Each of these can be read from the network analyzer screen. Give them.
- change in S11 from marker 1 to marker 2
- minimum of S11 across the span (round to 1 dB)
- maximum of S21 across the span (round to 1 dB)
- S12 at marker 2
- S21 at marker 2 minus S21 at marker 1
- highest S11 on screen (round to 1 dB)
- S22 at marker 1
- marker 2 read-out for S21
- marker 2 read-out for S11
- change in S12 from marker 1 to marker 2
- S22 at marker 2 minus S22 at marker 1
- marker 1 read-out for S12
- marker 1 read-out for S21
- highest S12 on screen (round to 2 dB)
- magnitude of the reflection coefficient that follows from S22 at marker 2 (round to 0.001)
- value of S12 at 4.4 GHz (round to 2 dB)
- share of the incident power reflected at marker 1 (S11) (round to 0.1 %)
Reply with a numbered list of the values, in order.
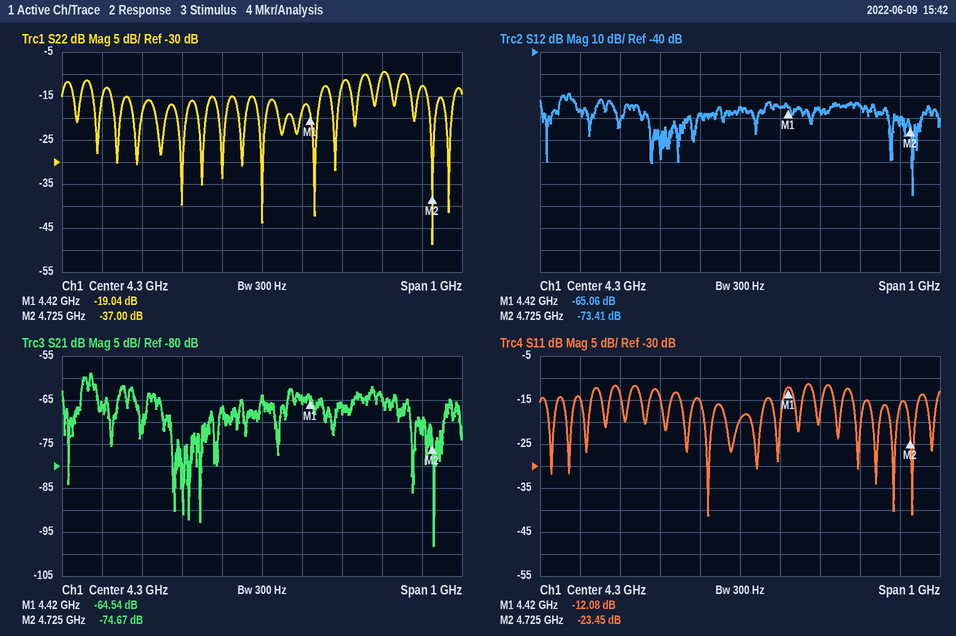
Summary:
1. -11.37 dB
2. -41 dB
3. -59 dB
4. -73.41 dB
5. -10.13 dB
6. -11 dB
7. -19.04 dB
8. -74.67 dB
9. -23.45 dB
10. -8.35 dB
11. -17.96 dB
12. -65.06 dB
13. -64.54 dB
14. -58 dB
15. 0.014
16. -66 dB
17. 6.2 %
